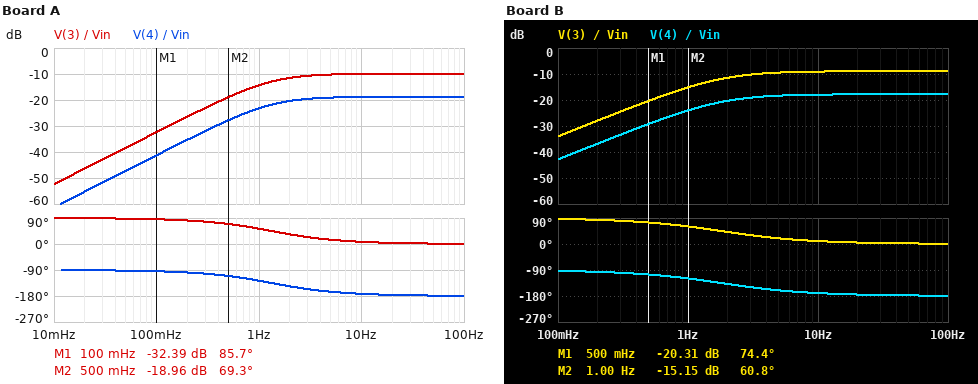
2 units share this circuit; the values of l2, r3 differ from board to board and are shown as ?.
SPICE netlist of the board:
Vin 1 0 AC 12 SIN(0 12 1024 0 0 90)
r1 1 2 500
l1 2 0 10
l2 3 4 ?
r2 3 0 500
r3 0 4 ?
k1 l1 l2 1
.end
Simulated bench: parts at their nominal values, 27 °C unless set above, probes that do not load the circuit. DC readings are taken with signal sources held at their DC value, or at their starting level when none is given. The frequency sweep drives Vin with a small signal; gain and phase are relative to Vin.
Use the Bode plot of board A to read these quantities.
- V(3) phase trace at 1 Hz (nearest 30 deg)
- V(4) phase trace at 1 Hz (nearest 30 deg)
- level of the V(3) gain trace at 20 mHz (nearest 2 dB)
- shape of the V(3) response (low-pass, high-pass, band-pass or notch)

60 deg
-120 deg
-46 dB
high-pass
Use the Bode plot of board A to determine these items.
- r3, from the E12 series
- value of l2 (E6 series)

180 Ω
68 H
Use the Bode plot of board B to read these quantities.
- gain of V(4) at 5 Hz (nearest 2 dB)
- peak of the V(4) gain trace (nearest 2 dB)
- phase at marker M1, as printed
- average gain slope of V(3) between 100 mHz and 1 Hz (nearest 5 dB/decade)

-18 dB
-18 dB
74.4 deg
20 dB/decade
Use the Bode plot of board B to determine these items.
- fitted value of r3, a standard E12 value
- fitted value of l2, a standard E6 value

180 Ω
47 H
